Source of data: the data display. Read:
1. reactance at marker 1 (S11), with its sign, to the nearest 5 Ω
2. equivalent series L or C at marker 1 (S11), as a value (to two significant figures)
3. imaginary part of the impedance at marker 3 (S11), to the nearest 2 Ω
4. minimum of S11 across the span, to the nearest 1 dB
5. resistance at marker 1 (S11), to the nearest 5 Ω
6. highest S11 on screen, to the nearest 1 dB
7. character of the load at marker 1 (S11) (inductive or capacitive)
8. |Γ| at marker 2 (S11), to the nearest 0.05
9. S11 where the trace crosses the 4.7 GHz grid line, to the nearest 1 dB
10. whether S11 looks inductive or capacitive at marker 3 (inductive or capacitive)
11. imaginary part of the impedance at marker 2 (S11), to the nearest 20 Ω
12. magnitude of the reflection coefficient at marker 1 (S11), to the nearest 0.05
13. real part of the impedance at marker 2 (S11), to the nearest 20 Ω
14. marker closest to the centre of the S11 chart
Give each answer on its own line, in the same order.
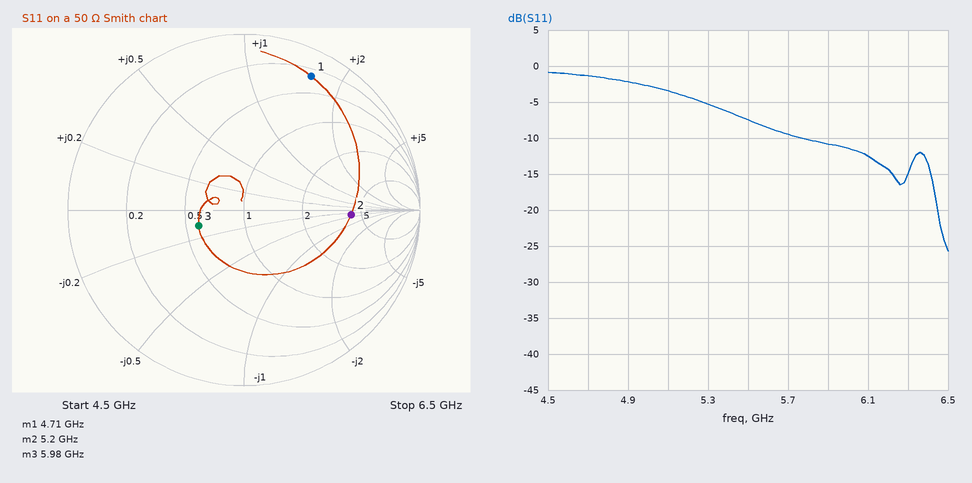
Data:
+80 Ω
2.7 nH
-6 Ω
-26 dB
15 Ω
-1 dB
inductive
0.60
-1 dB
capacitive
-20 Ω
0.85
200 Ω
marker 3
